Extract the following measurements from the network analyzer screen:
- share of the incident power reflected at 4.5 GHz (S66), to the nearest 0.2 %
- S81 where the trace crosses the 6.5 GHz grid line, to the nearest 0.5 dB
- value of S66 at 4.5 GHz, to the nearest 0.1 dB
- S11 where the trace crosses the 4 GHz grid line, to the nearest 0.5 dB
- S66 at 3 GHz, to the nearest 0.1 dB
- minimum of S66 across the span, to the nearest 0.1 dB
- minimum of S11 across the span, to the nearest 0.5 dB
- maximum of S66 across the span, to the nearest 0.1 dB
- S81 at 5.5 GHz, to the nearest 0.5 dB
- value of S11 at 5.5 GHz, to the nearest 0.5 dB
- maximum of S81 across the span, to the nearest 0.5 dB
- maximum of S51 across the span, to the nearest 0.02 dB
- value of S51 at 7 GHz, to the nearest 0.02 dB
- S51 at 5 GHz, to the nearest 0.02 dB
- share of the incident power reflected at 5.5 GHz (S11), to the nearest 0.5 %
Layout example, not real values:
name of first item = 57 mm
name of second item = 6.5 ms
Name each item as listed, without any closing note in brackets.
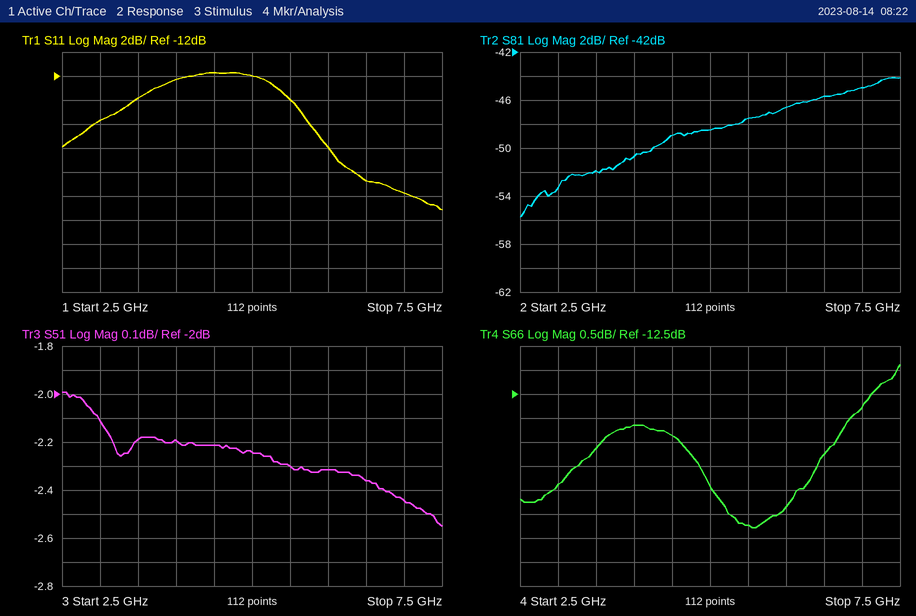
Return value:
share of the incident power reflected at 4.5 GHz (S66), to the nearest 0.2 % = 4.6 %
S81 where the trace crosses the 6.5 GHz grid line, to the nearest 0.5 dB = -45.5 dB
value of S66 at 4.5 GHz, to the nearest 0.1 dB = -13.4 dB
S11 where the trace crosses the 4 GHz grid line, to the nearest 0.5 dB = -12.5 dB
S66 at 3 GHz, to the nearest 0.1 dB = -14.4 dB
minimum of S66 across the span, to the nearest 0.1 dB = -15.3 dB
minimum of S11 across the span, to the nearest 0.5 dB = -23.0 dB
maximum of S66 across the span, to the nearest 0.1 dB = -11.9 dB
S81 at 5.5 GHz, to the nearest 0.5 dB = -47.5 dB
value of S11 at 5.5 GHz, to the nearest 0.5 dB = -14.0 dB
maximum of S81 across the span, to the nearest 0.5 dB = -44.0 dB
maximum of S51 across the span, to the nearest 0.02 dB = -2.00 dB
value of S51 at 7 GHz, to the nearest 0.02 dB = -2.44 dB
S51 at 5 GHz, to the nearest 0.02 dB = -2.24 dB
share of the incident power reflected at 5.5 GHz (S11), to the nearest 0.5 % = 4.0 %
